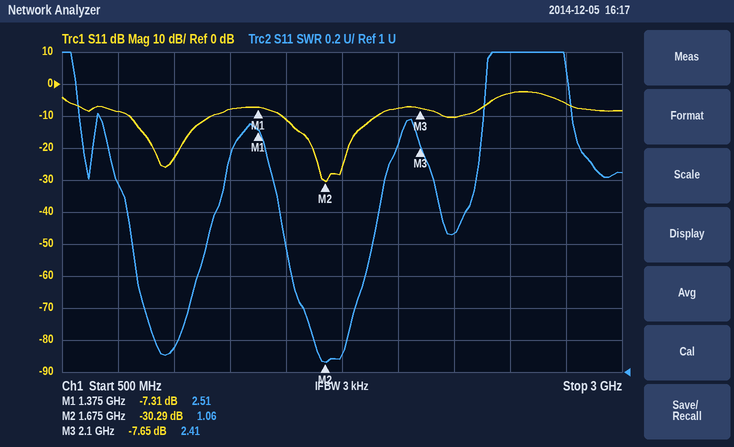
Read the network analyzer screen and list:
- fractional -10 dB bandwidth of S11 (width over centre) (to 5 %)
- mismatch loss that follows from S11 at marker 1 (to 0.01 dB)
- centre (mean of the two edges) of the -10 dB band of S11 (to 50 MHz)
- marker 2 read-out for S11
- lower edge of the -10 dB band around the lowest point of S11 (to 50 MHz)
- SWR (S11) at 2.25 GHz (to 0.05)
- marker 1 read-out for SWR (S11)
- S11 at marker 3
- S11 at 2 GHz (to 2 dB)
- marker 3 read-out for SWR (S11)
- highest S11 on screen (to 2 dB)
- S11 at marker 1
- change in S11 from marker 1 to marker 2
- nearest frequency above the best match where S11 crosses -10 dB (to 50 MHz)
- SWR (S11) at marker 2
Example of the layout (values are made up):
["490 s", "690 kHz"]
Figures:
["25 %", "0.89 dB", "1.70 GHz", "-30.29 dB", "1.50 GHz", "1.85", "2.51", "-7.65 dB", "-8 dB", "2.41", "-2 dB", "-7.31 dB", "-22.98 dB", "1.90 GHz", "1.06"]
